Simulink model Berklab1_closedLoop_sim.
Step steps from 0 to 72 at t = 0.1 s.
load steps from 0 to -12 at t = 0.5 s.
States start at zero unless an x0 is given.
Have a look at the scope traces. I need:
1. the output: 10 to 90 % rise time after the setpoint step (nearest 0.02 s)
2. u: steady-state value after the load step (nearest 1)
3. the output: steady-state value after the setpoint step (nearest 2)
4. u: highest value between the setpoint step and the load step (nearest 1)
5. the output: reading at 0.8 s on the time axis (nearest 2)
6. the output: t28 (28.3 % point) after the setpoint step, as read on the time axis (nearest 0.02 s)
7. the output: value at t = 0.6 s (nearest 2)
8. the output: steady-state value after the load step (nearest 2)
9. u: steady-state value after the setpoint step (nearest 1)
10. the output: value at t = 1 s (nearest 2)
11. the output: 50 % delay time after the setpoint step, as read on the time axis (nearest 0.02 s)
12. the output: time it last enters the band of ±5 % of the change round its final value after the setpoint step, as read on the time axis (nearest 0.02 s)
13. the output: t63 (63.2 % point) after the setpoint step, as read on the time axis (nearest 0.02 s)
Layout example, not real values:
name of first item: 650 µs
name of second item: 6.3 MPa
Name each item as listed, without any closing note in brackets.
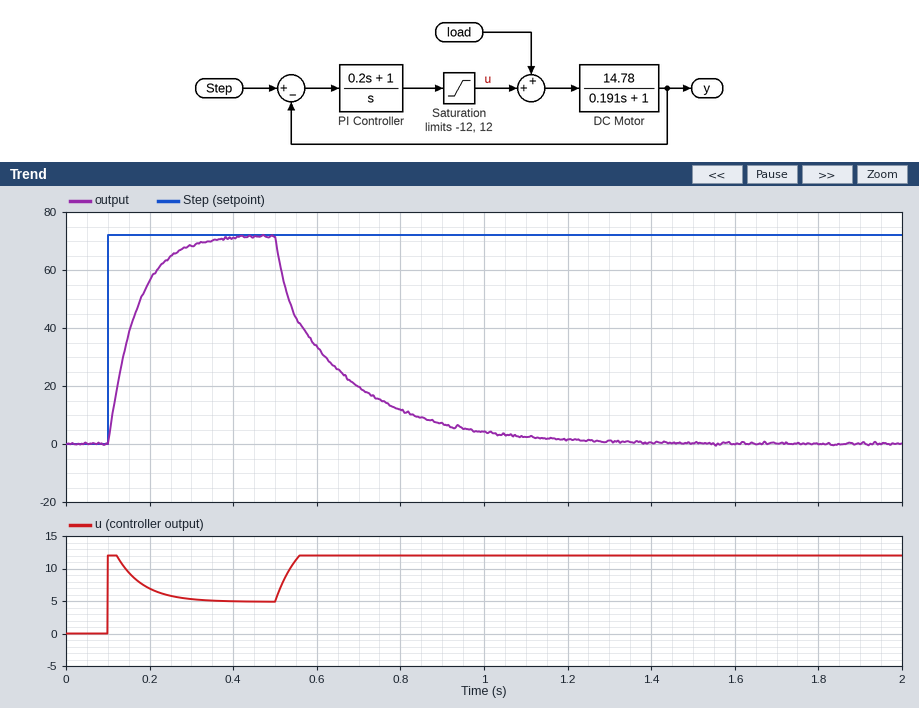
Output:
the output: 10 to 90 % rise time after the setpoint step: 0.14 s
u: steady-state value after the load step: 12
the output: steady-state value after the setpoint step: 72
u: highest value between the setpoint step and the load step: 12
the output: reading at 0.8 s on the time axis: 12
the output: t28 (28.3 % point) after the setpoint step, as read on the time axis: 0.12 s
the output: value at t = 0.6 s: 34
the output: steady-state value after the load step: 0
u: steady-state value after the setpoint step: 5
the output: value at t = 1 s: 4
the output: 50 % delay time after the setpoint step, as read on the time axis: 0.14 s
the output: time it last enters the band of ±5 % of the change round its final value after the setpoint step, as read on the time axis: 0.30 s
the output: t63 (63.2 % point) after the setpoint step, as read on the time axis: 0.16 s
